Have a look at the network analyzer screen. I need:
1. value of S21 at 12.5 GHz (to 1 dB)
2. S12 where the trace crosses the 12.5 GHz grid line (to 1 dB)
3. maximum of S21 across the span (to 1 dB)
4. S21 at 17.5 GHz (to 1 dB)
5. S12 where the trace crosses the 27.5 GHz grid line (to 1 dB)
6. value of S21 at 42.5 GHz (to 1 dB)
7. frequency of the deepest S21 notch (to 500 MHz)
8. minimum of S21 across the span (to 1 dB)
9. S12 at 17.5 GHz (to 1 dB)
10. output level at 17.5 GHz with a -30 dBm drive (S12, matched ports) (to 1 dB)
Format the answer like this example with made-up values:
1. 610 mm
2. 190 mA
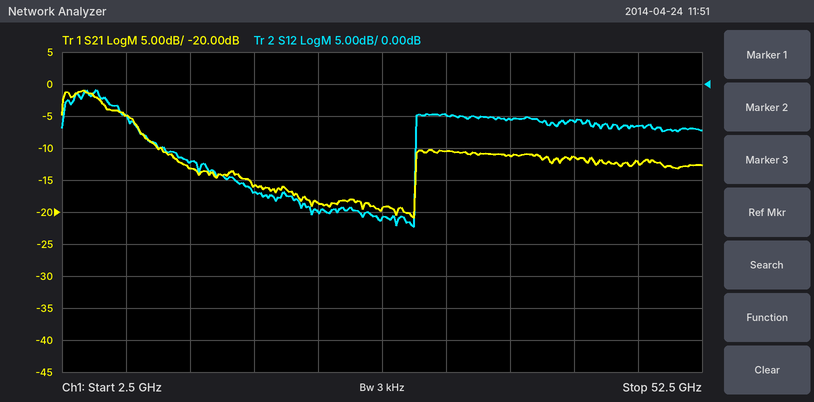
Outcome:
1. -13 dB
2. -12 dB
3. -1 dB
4. -16 dB
5. -21 dB
6. -11 dB
7. 30.0 GHz
8. -21 dB
9. -17 dB
10. -47 dBm
